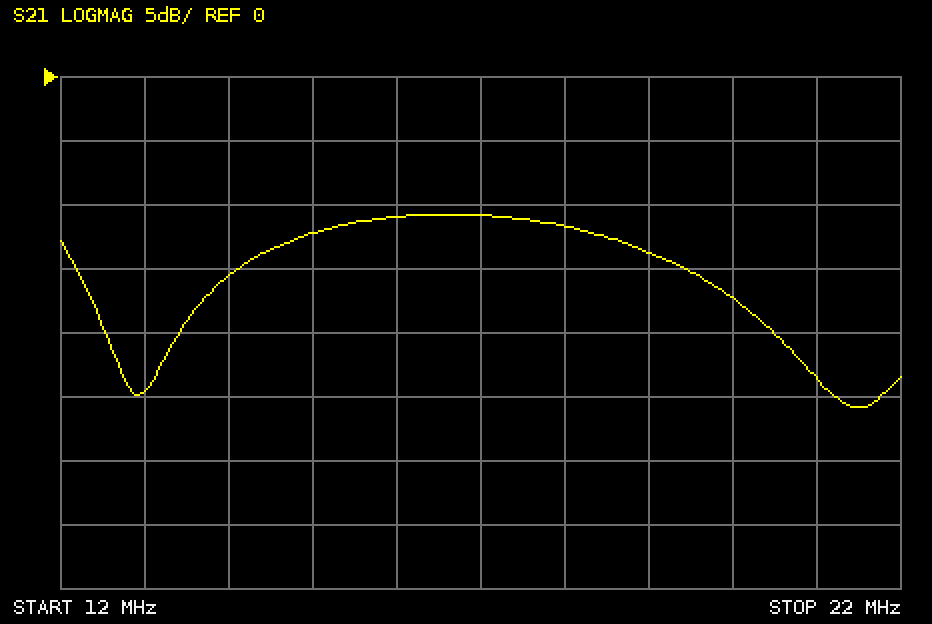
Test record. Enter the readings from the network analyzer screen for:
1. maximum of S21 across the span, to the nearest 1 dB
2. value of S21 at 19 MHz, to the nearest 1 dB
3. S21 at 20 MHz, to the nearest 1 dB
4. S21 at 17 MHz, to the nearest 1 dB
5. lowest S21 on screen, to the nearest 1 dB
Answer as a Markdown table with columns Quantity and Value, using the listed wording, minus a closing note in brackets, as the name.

| Quantity | Value |
|---|---|
| maximum of S21 across the span, to the nearest 1 dB | -11 dB |
| value of S21 at 19 MHz, to the nearest 1 dB | -14 dB |
| S21 at 20 MHz, to the nearest 1 dB | -17 dB |
| S21 at 17 MHz, to the nearest 1 dB | -11 dB |
| lowest S21 on screen, to the nearest 1 dB | -26 dB |
